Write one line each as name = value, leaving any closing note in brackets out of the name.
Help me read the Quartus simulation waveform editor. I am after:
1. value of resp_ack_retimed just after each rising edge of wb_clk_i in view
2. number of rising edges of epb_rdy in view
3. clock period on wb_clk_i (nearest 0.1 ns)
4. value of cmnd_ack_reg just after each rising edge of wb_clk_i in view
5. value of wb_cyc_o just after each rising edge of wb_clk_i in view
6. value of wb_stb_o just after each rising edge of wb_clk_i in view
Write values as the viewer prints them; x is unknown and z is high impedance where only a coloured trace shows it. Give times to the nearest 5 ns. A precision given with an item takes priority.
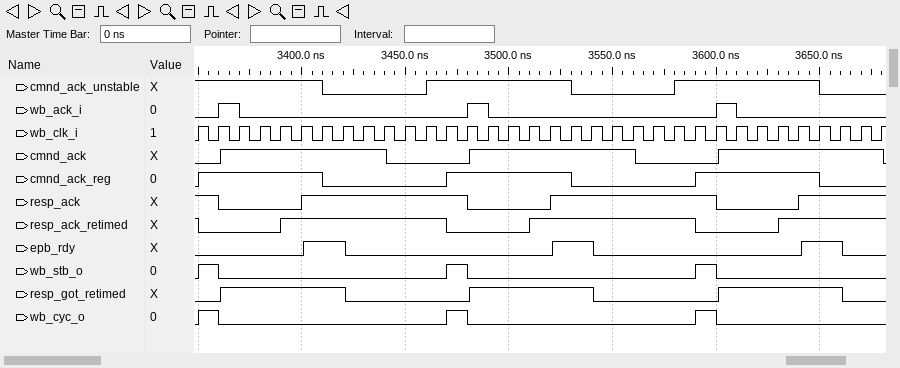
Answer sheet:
value of resp_ack_retimed just after each rising edge of wb_clk_i in view = 0 0 0 0 1 1 1 1 1 1 1 1 0 0 0 0 1 1 1 1 1 1 1 1 0 0 0 0 1 1 1 1 1 1
number of rising edges of epb_rdy in view = 3
clock period on wb_clk_i = 10 ns
value of cmnd_ack_reg just after each rising edge of wb_clk_i in view = 1 1 1 1 1 1 0 0 0 0 0 0 1 1 1 1 1 1 0 0 0 0 0 0 1 1 1 1 1 1 0 0 0 0
value of wb_cyc_o just after each rising edge of wb_clk_i in view = 1 0 0 0 0 0 0 0 0 0 0 0 1 0 0 0 0 0 0 0 0 0 0 0 1 0 0 0 0 0 0 0 0 0
value of wb_stb_o just after each rising edge of wb_clk_i in view = 1 0 0 0 0 0 0 0 0 0 0 0 1 0 0 0 0 0 0 0 0 0 0 0 1 0 0 0 0 0 0 0 0 0
